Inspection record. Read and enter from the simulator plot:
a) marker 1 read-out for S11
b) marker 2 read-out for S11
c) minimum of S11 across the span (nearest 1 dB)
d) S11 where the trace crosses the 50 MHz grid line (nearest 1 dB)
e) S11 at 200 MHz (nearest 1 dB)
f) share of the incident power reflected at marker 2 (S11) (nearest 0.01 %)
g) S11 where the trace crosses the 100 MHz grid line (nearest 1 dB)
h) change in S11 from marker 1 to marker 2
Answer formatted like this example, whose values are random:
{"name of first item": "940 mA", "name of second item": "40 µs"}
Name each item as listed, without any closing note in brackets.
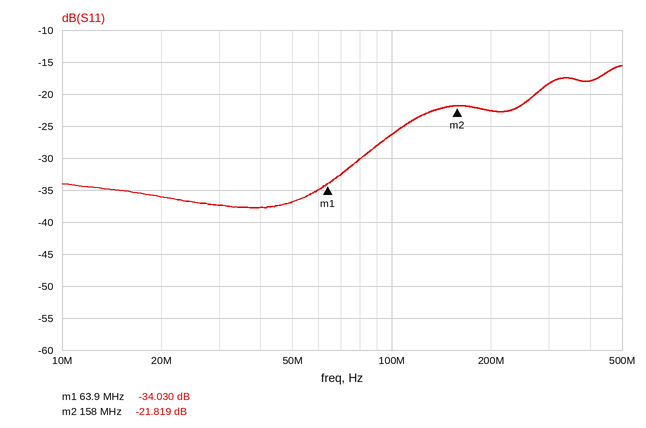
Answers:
{"marker 1 read-out for S11": "-34.030 dB", "marker 2 read-out for S11": "-21.819 dB", "minimum of S11 across the span": "-38 dB", "S11 where the trace crosses the 50 MHz grid line": "-37 dB", "S11 at 200 MHz": "-23 dB", "share of the incident power reflected at marker 2 (S11)": "0.66 %", "S11 where the trace crosses the 100 MHz grid line": "-26 dB", "change in S11 from marker 1 to marker 2": "12.211 dB"}
